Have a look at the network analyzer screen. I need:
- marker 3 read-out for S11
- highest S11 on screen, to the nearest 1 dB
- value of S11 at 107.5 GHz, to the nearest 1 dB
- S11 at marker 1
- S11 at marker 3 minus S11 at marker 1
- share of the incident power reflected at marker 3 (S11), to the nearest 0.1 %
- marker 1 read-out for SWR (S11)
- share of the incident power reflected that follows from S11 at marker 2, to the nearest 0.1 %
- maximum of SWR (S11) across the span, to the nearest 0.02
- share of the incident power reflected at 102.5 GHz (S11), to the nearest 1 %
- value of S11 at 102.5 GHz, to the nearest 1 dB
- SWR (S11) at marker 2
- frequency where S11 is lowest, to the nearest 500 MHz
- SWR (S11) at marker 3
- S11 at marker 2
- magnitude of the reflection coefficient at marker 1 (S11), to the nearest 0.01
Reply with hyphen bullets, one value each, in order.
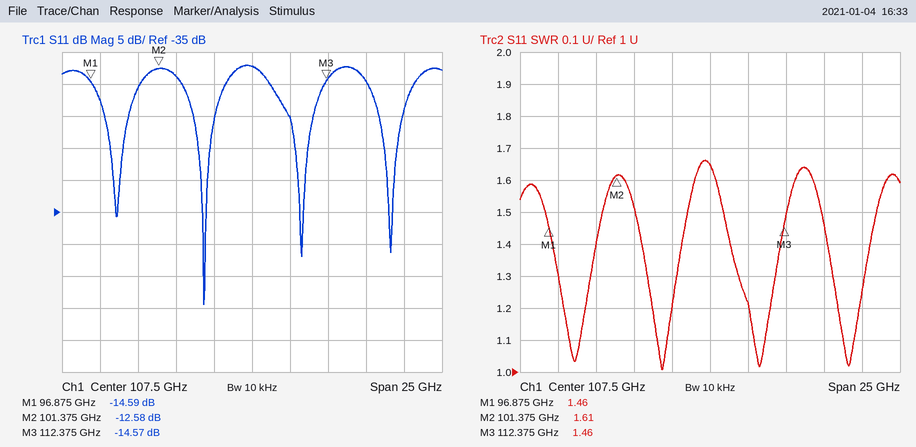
- -14.57 dB
- -12 dB
- -12 dB
- -14.59 dB
- 0.02 dB
- 3.5 %
- 1.46
- 5.5 %
- 1.66
- 4 %
- -14 dB
- 1.61
- 104.5 GHz
- 1.46
- -12.58 dB
- 0.19
